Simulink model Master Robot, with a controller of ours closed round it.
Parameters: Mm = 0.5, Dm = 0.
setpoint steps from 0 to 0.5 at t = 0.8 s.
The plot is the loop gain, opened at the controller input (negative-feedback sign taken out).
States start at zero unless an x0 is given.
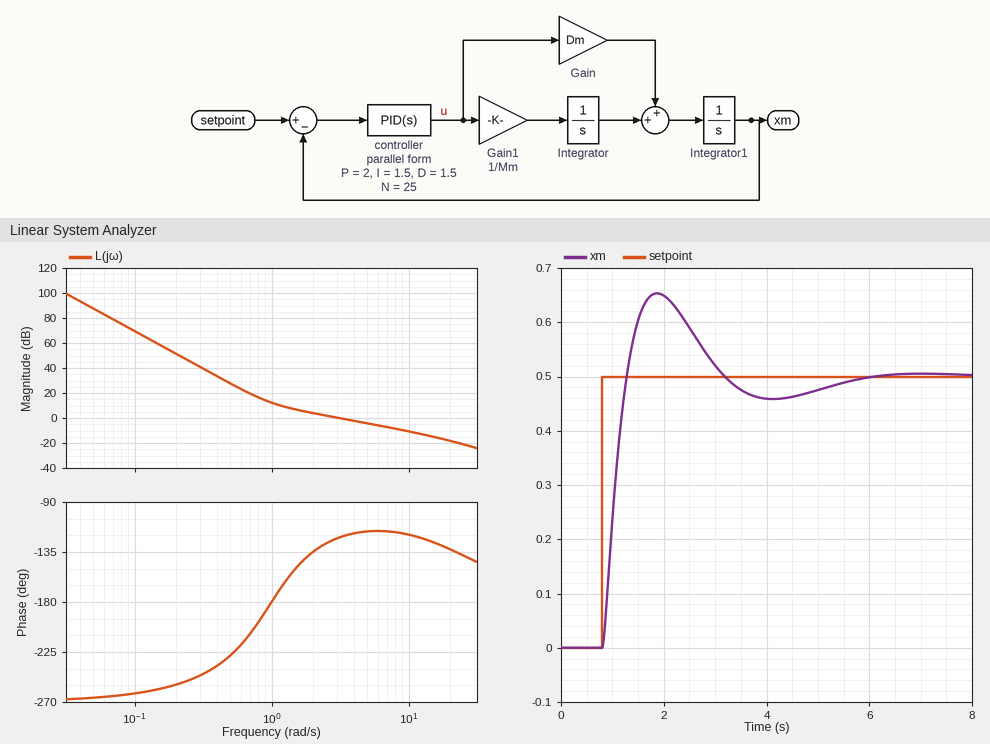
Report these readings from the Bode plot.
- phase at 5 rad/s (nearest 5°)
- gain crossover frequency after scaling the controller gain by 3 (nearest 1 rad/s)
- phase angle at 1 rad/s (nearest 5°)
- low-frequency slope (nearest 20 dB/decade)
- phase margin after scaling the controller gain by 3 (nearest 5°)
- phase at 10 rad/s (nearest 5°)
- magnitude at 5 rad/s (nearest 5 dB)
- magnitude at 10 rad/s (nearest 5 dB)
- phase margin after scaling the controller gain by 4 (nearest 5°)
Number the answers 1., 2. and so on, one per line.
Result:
1. -115°
2. 9 rad/s
3. -180°
4. -60 dB/decade
5. 60°
6. -120°
7. -5 dB
8. -10 dB
9. 60°
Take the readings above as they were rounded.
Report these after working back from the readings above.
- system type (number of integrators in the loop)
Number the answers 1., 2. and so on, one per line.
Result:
1. 3
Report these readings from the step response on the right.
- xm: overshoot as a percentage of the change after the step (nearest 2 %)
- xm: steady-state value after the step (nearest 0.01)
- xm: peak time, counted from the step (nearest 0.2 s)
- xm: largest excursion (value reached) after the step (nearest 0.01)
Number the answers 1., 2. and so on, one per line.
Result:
1. 30 %
2. 0.50
3. 1.0 s
4. 0.65
